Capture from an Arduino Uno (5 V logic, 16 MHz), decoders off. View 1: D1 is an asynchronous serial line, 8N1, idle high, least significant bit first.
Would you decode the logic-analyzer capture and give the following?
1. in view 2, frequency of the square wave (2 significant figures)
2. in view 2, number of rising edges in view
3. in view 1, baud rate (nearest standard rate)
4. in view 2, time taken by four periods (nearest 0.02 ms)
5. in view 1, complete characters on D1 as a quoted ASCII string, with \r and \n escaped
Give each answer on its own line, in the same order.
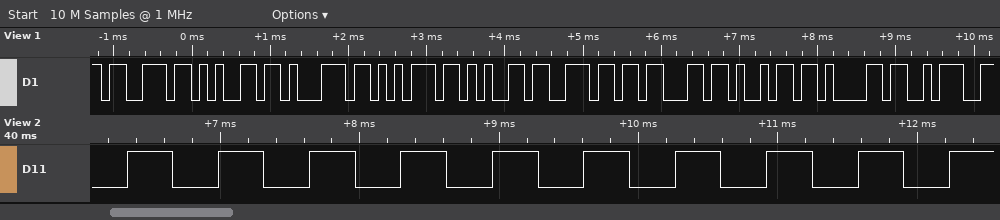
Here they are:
1.5 kHz
10
9600 baud
2.62 ms
"sequencia:"
